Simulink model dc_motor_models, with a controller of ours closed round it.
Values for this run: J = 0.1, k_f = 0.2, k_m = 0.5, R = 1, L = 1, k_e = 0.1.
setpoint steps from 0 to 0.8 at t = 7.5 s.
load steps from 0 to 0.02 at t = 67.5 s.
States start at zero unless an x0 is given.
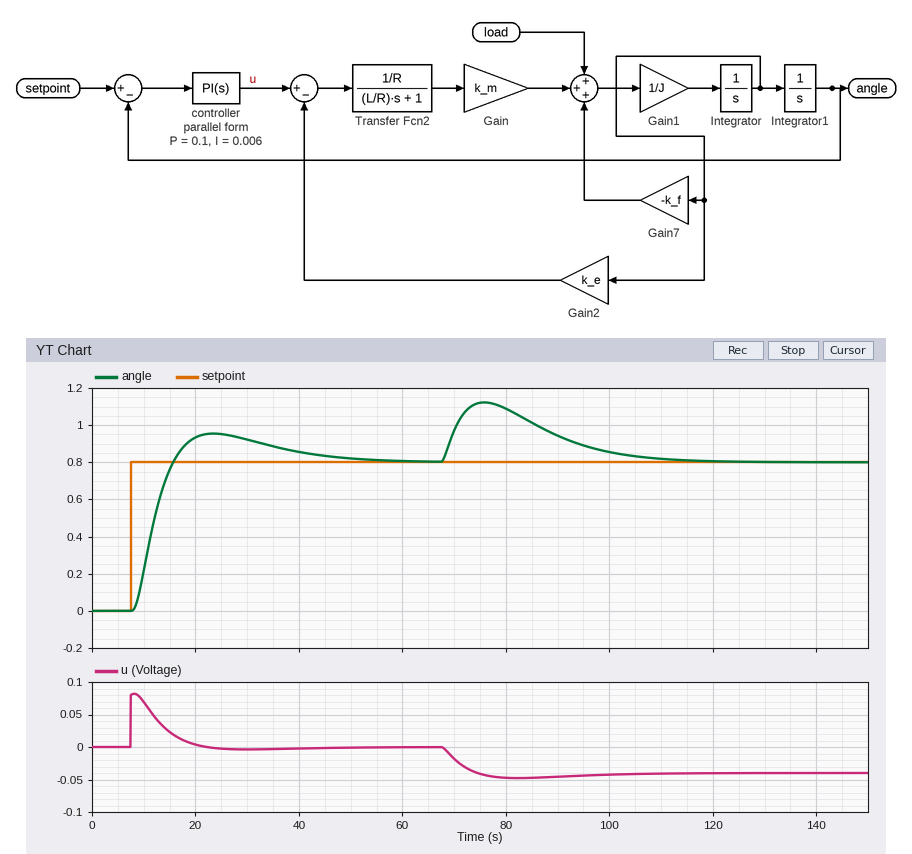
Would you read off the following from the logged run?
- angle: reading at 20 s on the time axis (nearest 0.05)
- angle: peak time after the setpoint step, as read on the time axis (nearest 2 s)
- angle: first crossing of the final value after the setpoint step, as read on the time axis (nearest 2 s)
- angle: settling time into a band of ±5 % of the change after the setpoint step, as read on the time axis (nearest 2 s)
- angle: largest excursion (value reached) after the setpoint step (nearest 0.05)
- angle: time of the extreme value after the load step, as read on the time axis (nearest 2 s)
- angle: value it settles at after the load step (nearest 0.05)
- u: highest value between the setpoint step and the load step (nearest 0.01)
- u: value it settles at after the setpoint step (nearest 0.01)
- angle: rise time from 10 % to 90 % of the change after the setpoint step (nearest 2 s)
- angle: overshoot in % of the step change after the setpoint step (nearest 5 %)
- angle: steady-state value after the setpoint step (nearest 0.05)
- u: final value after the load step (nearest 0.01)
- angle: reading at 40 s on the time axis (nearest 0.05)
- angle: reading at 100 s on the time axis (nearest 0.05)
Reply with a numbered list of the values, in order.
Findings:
1. 0.95
2. 24 s
3. 16 s
4. 44 s
5. 0.95
6. 76 s
7. 0.80
8. 0.08
9. 0.00
10. 6 s
11. 20 %
12. 0.80
13. -0.04
14. 0.85
15. 0.85
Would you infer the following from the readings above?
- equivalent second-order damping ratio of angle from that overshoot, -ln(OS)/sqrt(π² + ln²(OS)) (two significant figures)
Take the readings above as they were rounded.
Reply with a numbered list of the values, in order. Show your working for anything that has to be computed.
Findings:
1. ln(0.2) = -1.609; 1.609 / sqrt(9.870 + 2.590) = 0.46
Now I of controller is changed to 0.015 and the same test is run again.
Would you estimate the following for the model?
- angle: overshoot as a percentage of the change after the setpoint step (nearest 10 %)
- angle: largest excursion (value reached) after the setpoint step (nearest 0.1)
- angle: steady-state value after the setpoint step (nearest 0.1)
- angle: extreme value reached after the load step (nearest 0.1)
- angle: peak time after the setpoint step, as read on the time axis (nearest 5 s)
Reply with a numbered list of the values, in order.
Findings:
1. 40 %
2. 1.1
3. 0.8
4. 1.1
5. 20 s
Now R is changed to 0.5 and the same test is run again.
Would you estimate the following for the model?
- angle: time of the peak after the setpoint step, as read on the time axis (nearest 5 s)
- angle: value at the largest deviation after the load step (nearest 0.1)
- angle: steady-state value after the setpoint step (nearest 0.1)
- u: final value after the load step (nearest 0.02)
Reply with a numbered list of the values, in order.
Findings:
1. 15 s
2. 1.0
3. 0.8
4. -0.02
